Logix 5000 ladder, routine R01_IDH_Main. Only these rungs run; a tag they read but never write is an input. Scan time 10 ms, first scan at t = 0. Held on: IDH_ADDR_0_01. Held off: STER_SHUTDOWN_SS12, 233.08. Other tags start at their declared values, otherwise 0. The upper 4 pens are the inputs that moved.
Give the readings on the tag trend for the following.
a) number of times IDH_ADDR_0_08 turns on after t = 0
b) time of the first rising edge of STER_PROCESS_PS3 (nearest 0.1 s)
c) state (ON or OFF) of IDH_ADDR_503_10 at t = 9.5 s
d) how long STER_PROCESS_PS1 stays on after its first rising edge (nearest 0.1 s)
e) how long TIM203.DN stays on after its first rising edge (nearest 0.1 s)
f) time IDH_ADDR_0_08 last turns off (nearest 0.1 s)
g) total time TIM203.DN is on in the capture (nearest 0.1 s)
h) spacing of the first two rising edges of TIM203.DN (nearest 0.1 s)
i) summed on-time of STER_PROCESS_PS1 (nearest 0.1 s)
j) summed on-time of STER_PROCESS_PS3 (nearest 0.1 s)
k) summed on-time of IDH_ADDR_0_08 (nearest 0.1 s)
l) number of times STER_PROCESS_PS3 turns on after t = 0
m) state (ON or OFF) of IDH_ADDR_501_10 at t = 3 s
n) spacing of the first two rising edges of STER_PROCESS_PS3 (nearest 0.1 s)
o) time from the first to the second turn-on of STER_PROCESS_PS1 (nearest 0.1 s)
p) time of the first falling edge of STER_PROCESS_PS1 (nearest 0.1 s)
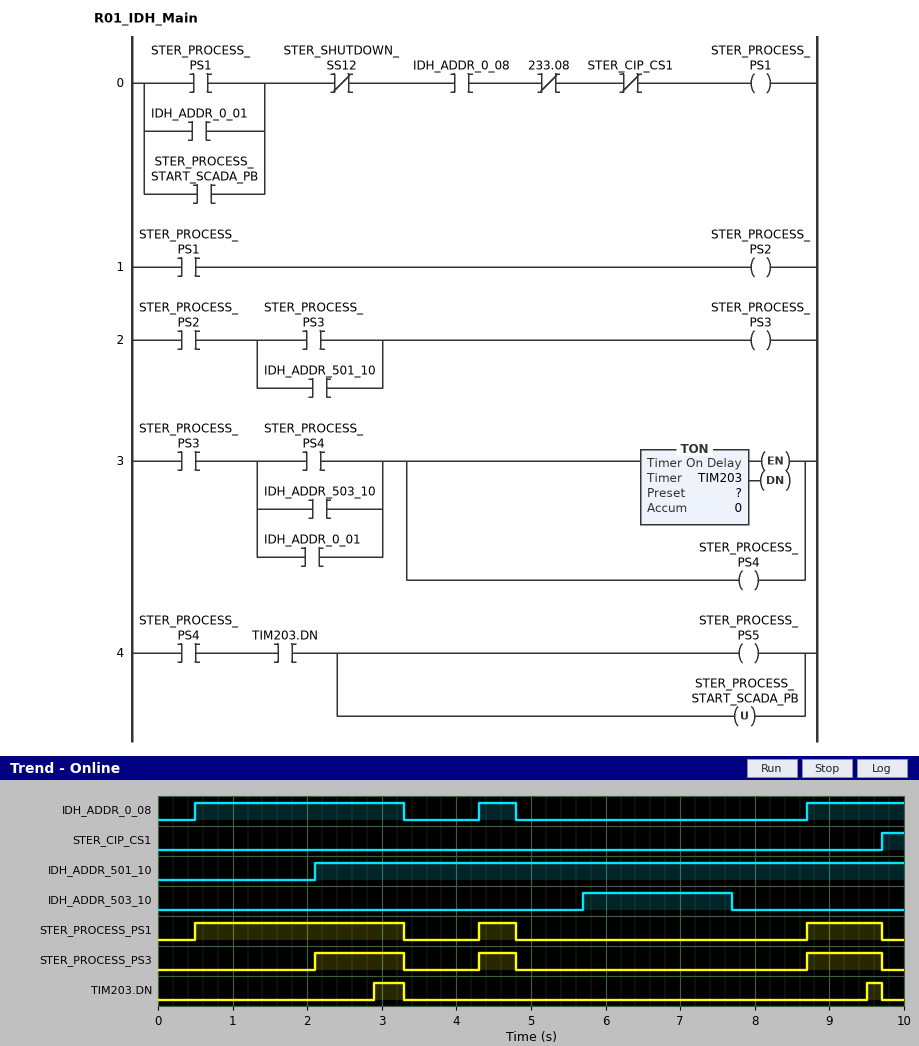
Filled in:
3
2.1 s
OFF
2.8 s
0.4 s
4.8 s
0.6 s
6.6 s
4.3 s
2.7 s
4.6 s
3
ON
2.2 s
3.8 s
3.3 s
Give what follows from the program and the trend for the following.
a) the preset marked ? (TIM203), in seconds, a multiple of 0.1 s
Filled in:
0.8 s
